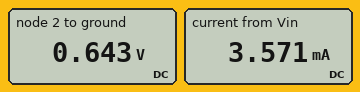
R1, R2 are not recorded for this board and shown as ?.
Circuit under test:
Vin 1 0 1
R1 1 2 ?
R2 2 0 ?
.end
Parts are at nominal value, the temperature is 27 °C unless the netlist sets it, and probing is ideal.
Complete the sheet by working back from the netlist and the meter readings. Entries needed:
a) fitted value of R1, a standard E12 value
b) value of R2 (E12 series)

100 Ω
180 Ω
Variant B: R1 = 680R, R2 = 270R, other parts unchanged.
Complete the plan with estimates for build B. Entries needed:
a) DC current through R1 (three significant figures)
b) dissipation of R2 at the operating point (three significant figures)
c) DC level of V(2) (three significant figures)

1.05 mA
299 µW
284 mV
